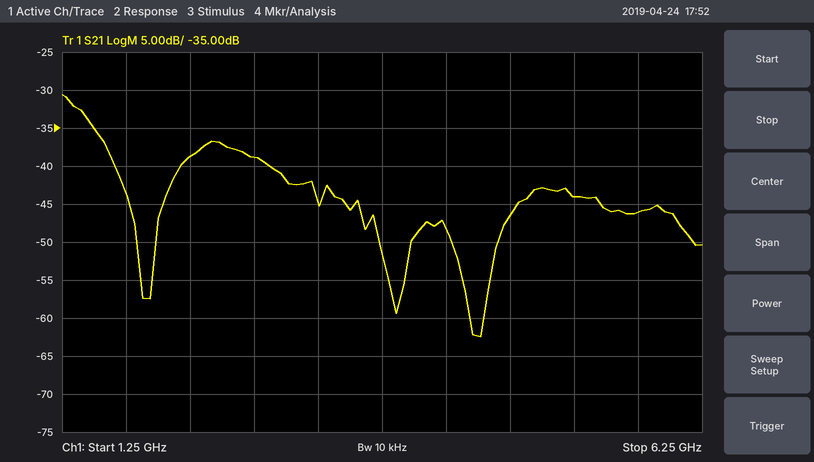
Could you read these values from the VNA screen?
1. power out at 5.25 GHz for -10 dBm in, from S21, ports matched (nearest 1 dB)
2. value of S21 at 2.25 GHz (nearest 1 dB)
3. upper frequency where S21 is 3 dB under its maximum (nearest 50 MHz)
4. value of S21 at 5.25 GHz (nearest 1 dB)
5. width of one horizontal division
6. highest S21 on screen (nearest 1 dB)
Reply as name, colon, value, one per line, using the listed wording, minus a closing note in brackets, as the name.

power out at 5.25 GHz for -10 dBm in, from S21, ports matched: -54 dBm
value of S21 at 2.25 GHz: -39 dB
upper frequency where S21 is 3 dB under its maximum: 1.45 GHz
value of S21 at 5.25 GHz: -44 dB
width of one horizontal division: 500 MHz
highest S21 on screen: -31 dB
